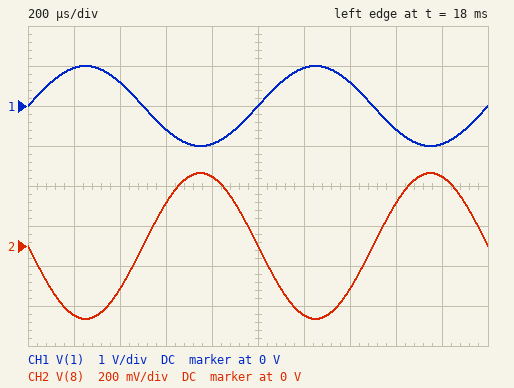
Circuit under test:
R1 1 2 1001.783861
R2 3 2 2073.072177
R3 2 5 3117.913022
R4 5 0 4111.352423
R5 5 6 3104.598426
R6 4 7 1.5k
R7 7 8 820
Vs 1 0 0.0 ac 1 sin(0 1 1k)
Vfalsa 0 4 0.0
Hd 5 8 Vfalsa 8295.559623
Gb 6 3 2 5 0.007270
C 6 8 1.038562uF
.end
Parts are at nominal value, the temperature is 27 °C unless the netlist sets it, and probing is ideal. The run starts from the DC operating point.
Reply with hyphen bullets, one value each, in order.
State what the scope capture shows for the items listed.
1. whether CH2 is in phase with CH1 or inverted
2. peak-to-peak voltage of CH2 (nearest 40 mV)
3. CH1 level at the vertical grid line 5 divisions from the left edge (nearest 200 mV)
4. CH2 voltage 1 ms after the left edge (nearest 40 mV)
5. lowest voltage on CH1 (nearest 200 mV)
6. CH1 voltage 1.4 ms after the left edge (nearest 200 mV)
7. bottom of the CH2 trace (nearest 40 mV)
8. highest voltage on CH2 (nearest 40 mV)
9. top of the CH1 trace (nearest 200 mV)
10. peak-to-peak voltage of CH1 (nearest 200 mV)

- inverted
- 720 mV
- 0 V
- 0 V
- -1.0 V
- 600 mV
- -360 mV
- 360 mV
- 1.0 V
- 2.0 V
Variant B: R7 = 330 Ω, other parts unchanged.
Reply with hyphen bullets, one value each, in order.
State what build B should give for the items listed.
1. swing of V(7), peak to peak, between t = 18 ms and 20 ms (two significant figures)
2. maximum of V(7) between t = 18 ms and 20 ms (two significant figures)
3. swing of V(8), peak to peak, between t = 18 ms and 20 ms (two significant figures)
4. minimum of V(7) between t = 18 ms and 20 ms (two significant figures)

- 430 mV
- 220 mV
- 530 mV
- -220 mV
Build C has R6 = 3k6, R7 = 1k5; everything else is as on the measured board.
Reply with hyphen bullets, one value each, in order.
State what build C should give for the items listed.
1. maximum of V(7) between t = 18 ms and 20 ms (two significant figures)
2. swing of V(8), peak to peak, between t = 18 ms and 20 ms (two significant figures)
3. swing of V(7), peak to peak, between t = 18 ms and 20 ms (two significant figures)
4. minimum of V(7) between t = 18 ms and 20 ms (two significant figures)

- 1.2 V
- 3.4 V
- 2.4 V
- -1.2 V
